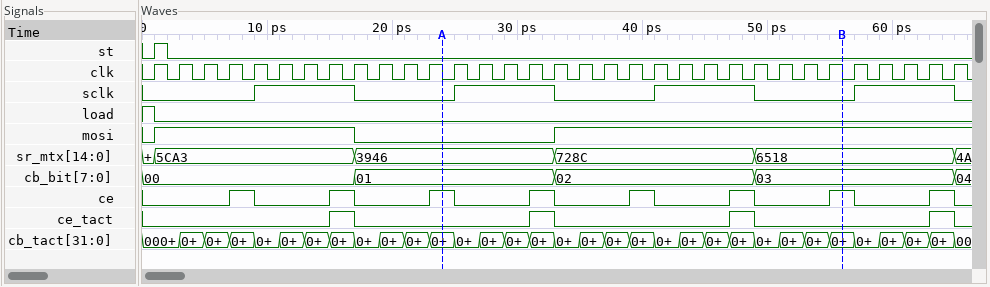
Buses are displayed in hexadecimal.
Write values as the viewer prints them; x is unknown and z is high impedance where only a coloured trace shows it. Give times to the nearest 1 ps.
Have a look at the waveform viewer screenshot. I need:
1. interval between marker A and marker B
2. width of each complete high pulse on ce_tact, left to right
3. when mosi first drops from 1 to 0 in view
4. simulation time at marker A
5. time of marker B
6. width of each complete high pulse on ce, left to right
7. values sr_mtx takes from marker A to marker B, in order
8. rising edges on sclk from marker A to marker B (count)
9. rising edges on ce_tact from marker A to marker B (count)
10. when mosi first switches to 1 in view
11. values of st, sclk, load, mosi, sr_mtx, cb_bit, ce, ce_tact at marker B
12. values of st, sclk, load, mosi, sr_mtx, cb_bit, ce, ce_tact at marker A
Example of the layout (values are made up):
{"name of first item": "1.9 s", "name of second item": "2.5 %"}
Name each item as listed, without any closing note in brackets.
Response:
{"interval between marker A and marker B": "32 ps", "width of each complete high pulse on ce_tact, left to right": "2 ps, 2 ps, 2 ps, 2 ps", "when mosi first drops from 1 to 0 in view": "17 ps", "simulation time at marker A": "24 ps", "time of marker B": "56 ps", "width of each complete high pulse on ce, left to right": "2 ps, 2 ps, 2 ps, 2 ps, 2 ps, 2 ps, 2 ps, 2 ps", "values sr_mtx takes from marker A to marker B, in order": "3946, 728C, 6518", "rising edges on sclk from marker A to marker B": "2", "rising edges on ce_tact from marker A to marker B": "2", "when mosi first switches to 1 in view": "1 ps", "values of st, sclk, load, mosi, sr_mtx, cb_bit, ce, ce_tact at marker B": "st=0, sclk=0, load=0, mosi=1, sr_mtx=6518, cb_bit=03, ce=1, ce_tact=0", "values of st, sclk, load, mosi, sr_mtx, cb_bit, ce, ce_tact at marker A": "st=0, sclk=0, load=0, mosi=0, sr_mtx=3946, cb_bit=01, ce=1, ce_tact=0"}
